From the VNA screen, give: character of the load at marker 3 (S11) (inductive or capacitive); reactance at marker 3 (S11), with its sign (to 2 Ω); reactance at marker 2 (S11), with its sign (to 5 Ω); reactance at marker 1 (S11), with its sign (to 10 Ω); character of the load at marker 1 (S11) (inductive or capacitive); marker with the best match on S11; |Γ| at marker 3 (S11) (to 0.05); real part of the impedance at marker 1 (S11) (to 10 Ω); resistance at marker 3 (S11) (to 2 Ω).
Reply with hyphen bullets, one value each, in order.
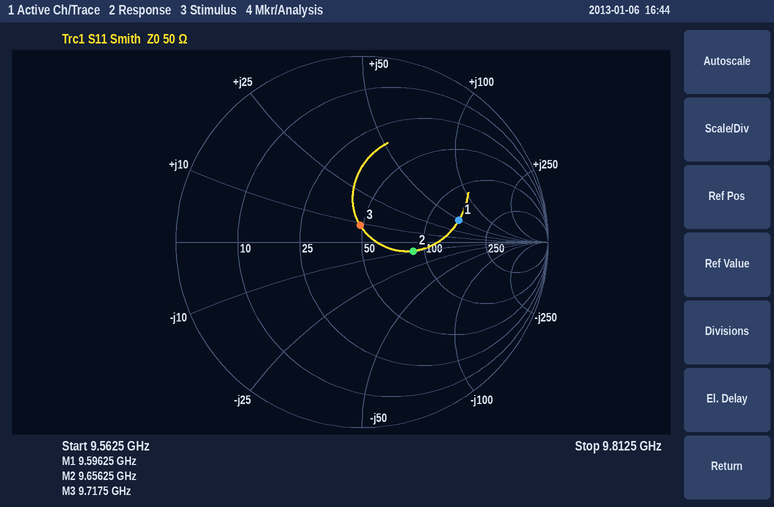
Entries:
- inductive
- +8 Ω
- -10 Ω
- +50 Ω
- inductive
- marker 3
- 0.10
- 150 Ω
- 48 Ω
